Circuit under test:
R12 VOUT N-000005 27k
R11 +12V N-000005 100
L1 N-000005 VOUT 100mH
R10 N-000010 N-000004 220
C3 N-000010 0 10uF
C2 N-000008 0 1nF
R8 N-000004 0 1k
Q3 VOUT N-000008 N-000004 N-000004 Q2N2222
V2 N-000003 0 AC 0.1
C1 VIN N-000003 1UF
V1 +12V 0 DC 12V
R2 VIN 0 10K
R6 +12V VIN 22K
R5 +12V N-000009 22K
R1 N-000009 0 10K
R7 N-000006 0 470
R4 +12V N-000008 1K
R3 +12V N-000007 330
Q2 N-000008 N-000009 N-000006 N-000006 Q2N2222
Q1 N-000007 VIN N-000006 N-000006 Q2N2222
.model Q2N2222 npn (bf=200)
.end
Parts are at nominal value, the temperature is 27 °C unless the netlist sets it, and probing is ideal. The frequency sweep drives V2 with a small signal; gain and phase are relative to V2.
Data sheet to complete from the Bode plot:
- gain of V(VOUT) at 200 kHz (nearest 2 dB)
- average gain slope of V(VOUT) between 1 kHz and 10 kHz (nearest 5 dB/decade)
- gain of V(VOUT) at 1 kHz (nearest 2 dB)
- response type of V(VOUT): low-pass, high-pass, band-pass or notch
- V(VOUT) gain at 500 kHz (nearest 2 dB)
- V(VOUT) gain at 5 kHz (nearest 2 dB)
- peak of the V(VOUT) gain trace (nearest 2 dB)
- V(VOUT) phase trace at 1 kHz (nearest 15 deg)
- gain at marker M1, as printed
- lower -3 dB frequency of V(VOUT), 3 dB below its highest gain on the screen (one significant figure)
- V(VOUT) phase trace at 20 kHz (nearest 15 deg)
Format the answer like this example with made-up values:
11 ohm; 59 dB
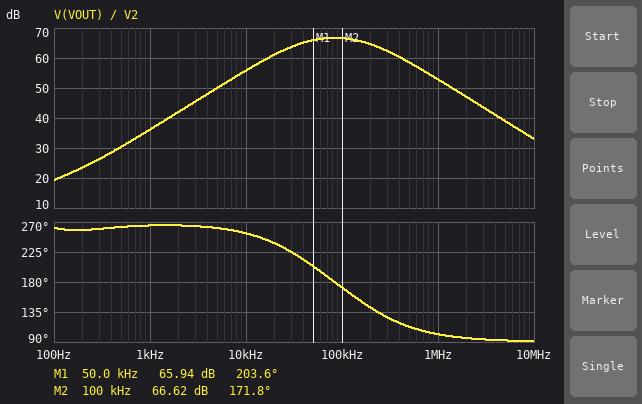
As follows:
64 dB; 20 dB/decade; 36 dB; band-pass; 58 dB; 50 dB; 66 dB; 270 deg; 65.94 dB; 30 kHz; 240 deg
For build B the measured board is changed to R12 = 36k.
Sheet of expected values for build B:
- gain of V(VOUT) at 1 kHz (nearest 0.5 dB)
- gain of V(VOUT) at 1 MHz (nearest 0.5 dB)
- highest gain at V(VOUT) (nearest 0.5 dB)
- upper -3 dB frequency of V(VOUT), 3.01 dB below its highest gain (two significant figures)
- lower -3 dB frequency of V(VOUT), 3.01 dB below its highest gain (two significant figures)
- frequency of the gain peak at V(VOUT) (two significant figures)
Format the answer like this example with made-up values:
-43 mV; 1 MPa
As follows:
36.0 dB; 55.5 dB; 68.5 dB; 260 kHz; 36 kHz; 97 kHz
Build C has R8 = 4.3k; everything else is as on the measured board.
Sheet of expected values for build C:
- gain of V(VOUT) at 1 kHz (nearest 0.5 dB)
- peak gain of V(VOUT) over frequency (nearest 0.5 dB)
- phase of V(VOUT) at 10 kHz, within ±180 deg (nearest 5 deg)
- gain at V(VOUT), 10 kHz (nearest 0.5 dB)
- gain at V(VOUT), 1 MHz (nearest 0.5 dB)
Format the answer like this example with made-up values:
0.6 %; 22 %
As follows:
34.5 dB; 65.0 dB; -105 deg; 54.0 dB; 51.0 dB
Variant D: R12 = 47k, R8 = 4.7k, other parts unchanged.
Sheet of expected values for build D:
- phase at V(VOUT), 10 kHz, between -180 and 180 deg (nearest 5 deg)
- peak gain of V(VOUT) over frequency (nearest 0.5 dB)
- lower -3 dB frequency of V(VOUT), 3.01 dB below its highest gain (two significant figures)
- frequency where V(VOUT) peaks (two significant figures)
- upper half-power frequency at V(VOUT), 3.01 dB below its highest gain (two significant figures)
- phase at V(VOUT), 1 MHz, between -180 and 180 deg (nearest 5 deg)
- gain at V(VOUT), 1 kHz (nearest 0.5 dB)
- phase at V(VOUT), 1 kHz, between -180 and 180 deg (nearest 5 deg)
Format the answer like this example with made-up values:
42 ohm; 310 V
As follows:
-100 deg; 68.5 dB; 43 kHz; 110 kHz; 280 kHz; 105 deg; 34.5 dB; -95 deg
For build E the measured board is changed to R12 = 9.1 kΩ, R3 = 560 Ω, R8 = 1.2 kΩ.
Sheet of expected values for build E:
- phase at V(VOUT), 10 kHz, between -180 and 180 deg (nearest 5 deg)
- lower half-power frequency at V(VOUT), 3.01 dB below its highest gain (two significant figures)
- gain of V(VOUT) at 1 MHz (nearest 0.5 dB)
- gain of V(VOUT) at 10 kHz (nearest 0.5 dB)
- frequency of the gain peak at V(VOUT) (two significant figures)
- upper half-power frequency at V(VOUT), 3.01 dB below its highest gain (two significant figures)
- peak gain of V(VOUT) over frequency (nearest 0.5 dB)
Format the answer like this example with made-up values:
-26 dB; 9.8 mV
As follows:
-130 deg; 12 kHz; 43.0 dB; 54.0 dB; 49 kHz; 190 kHz; 58.5 dB
